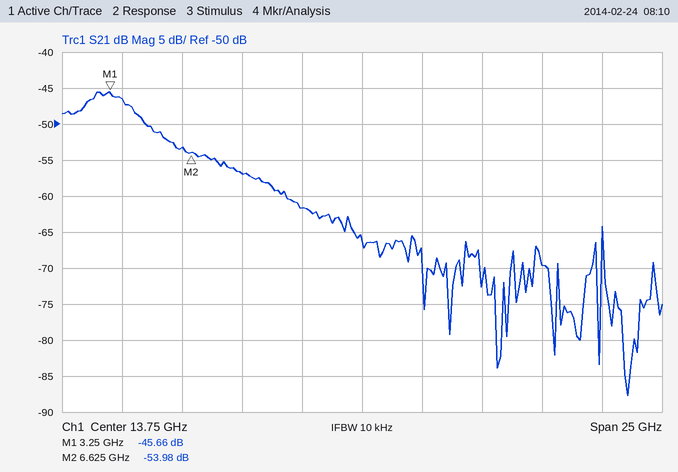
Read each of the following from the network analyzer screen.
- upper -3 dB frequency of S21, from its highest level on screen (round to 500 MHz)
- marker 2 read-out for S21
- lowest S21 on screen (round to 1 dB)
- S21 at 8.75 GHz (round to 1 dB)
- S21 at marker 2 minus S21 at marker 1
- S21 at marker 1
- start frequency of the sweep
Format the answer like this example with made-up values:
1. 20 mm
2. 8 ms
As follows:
1. 4.5 GHz
2. -53.98 dB
3. -88 dB
4. -57 dB
5. -8.32 dB
6. -45.66 dB
7. 1.25 GHz
